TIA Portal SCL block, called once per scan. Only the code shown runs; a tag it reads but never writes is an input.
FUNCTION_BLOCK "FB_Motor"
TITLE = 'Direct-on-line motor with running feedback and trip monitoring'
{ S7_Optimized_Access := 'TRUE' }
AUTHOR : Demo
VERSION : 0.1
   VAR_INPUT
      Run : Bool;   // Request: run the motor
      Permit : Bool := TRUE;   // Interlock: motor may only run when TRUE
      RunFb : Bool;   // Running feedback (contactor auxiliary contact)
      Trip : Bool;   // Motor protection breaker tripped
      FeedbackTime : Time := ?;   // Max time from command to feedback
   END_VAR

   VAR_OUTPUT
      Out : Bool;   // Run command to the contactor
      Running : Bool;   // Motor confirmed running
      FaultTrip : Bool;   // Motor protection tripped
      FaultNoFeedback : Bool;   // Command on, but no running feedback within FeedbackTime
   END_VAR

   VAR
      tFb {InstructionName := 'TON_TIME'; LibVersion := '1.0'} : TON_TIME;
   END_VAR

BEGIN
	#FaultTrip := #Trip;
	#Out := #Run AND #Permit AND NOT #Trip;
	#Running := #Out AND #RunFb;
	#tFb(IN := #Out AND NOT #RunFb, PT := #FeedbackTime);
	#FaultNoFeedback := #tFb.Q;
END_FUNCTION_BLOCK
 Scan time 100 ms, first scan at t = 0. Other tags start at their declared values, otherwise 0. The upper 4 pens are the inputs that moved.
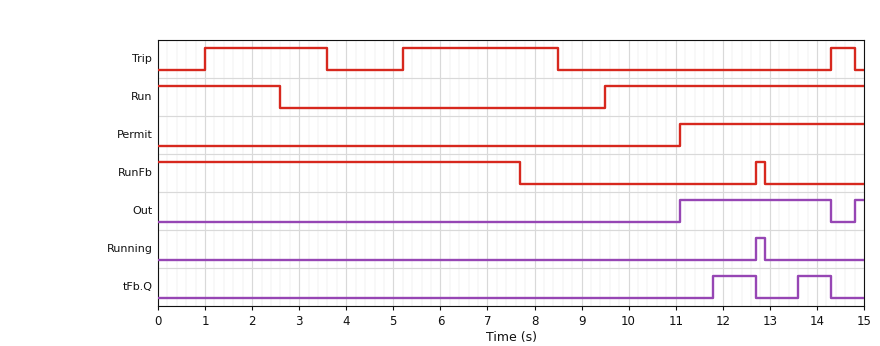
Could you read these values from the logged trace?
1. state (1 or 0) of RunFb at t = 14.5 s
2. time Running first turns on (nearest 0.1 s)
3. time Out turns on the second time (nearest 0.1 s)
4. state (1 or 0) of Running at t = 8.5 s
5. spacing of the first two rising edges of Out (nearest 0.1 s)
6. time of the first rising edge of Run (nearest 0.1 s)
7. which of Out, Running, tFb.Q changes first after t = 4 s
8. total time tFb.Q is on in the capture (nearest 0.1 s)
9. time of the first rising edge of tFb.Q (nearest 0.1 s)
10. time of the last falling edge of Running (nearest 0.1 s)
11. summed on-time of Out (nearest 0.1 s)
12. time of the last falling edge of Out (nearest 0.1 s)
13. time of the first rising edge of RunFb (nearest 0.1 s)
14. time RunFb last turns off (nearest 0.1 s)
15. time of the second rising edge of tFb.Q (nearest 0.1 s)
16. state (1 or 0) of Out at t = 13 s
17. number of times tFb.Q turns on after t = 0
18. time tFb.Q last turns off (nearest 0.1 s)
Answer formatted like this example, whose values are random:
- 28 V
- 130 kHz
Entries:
- 0
- 12.7 s
- 14.8 s
- 0
- 3.7 s
- 9.5 s
- Out
- 1.6 s
- 11.8 s
- 12.9 s
- 3.4 s
- 14.3 s
- 12.7 s
- 12.9 s
- 13.6 s
- 1
- 2
- 14.3 s
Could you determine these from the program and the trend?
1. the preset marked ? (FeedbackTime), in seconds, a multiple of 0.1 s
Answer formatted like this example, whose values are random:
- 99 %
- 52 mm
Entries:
- 0.7 s
